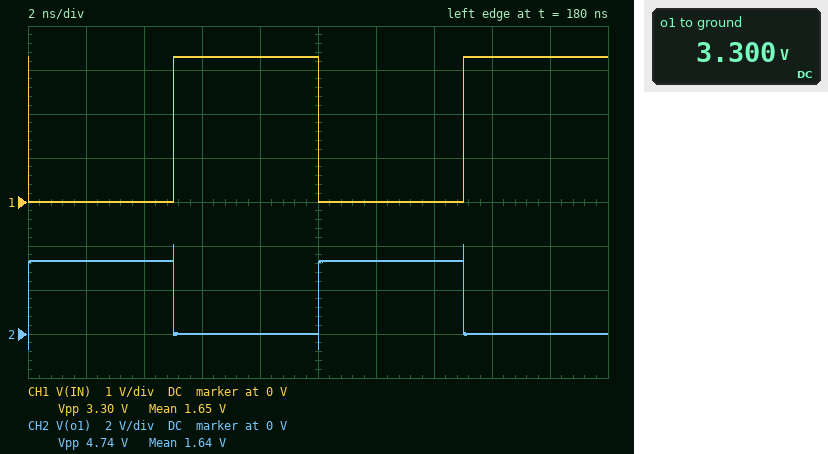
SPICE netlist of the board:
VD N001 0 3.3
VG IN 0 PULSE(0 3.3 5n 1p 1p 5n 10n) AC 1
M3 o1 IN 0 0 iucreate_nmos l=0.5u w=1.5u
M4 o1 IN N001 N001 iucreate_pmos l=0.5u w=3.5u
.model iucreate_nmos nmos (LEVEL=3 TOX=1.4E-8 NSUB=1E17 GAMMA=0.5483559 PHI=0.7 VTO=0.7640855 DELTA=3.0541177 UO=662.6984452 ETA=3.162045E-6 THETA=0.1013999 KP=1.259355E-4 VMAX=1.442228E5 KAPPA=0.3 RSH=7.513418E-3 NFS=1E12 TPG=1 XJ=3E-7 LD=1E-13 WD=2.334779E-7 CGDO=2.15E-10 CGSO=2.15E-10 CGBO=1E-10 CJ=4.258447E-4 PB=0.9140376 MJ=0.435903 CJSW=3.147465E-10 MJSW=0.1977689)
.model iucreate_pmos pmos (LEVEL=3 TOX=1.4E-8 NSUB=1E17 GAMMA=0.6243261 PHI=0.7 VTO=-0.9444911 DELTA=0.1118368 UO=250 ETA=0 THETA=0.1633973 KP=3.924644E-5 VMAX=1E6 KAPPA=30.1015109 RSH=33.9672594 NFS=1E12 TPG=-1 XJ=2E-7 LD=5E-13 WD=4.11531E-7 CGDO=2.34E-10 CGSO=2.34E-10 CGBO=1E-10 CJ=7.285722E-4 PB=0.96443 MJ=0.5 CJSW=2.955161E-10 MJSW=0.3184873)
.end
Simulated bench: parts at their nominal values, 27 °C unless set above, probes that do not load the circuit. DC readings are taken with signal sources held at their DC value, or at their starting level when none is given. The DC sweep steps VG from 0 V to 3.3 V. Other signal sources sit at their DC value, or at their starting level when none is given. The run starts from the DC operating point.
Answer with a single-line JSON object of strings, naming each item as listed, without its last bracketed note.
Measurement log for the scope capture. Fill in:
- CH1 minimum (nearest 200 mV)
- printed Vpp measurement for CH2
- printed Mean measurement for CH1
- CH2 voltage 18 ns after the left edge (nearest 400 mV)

{"CH1 minimum": "0 V", "printed Vpp measurement for CH2": "4.74 V", "printed Mean measurement for CH1": "1.65 V", "CH2 voltage 18 ns after the left edge": "0 V"}
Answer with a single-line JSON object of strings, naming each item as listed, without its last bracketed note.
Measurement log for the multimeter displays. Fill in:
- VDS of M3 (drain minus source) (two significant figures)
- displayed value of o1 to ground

{"VDS of M3 (drain minus source)": "3.3 V", "displayed value of o1 to ground": "3.300 V"}
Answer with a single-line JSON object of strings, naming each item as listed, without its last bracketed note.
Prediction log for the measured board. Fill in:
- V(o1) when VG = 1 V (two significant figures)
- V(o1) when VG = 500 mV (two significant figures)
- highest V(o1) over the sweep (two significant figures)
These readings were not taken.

{"V(o1) when VG = 1 V": "3.3 V", "V(o1) when VG = 500 mV": "3.3 V", "highest V(o1) over the sweep": "3.3 V"}
